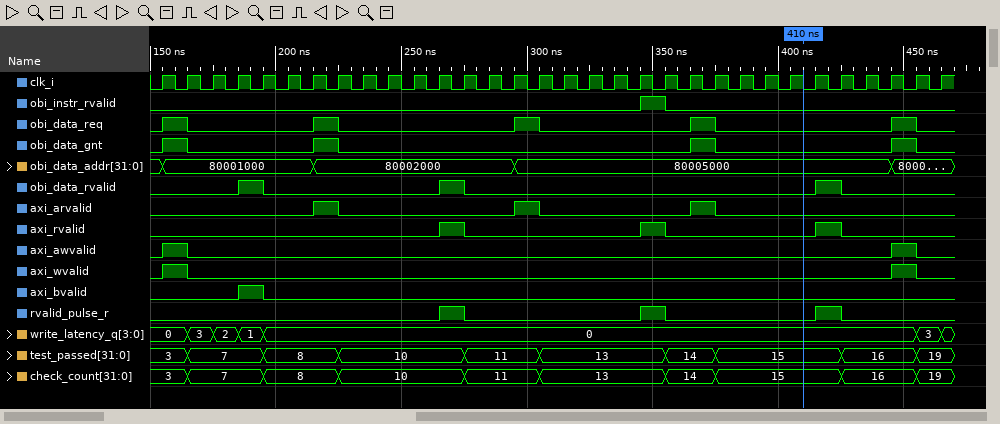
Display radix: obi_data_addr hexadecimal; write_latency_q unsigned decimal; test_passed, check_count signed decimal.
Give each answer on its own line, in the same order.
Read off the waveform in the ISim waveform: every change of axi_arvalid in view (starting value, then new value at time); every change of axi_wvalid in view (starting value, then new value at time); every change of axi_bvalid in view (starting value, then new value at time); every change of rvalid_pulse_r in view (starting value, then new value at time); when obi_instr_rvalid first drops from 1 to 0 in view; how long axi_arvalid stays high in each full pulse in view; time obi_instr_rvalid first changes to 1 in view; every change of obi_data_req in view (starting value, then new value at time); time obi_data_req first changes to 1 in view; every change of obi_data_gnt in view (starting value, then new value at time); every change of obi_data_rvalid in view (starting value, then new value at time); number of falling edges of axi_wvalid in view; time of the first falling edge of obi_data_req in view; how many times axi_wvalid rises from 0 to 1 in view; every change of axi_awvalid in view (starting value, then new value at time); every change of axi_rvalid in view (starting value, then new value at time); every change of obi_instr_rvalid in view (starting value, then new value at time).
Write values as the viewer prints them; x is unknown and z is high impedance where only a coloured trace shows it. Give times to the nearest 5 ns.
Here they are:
0, 1 at 215 ns, 0 at 225 ns, 1 at 295 ns, 0 at 305 ns, 1 at 365 ns, 0 at 375 ns
0, 1 at 155 ns, 0 at 165 ns, 1 at 445 ns, 0 at 455 ns
0, 1 at 185 ns, 0 at 195 ns
0, 1 at 265 ns, 0 at 275 ns, 1 at 345 ns, 0 at 355 ns, 1 at 415 ns, 0 at 425 ns
355 ns
10 ns, 10 ns, 10 ns
345 ns
0, 1 at 155 ns, 0 at 165 ns, 1 at 215 ns, 0 at 225 ns, 1 at 295 ns, 0 at 305 ns, 1 at 365 ns, 0 at 375 ns, 1 at 445 ns, 0 at 455 ns
155 ns
0, 1 at 155 ns, 0 at 165 ns, 1 at 215 ns, 0 at 225 ns, 1 at 365 ns, 0 at 375 ns, 1 at 445 ns, 0 at 455 ns
0, 1 at 185 ns, 0 at 195 ns, 1 at 265 ns, 0 at 275 ns, 1 at 415 ns, 0 at 425 ns
2
165 ns
2
0, 1 at 155 ns, 0 at 165 ns, 1 at 445 ns, 0 at 455 ns
0, 1 at 265 ns, 0 at 275 ns, 1 at 345 ns, 0 at 355 ns, 1 at 415 ns, 0 at 425 ns
0, 1 at 345 ns, 0 at 355 ns
